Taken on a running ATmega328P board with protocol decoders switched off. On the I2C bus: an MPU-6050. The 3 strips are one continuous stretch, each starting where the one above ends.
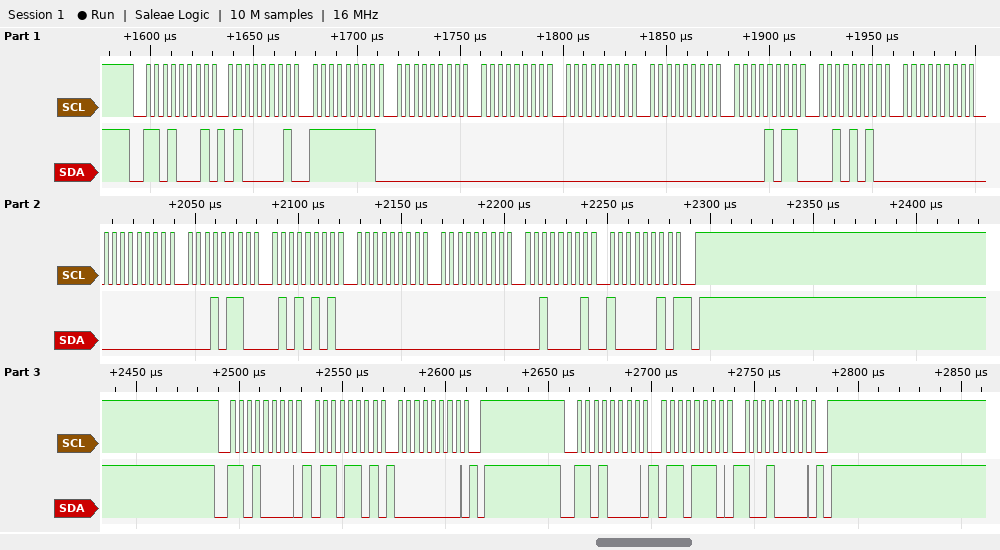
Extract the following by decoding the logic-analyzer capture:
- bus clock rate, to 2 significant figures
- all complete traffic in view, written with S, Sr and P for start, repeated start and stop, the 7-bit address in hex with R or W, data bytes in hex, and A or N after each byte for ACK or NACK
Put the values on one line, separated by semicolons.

250 kHz; S 68R A 41 A FF A 00 A 00 A 00 A 00 A 0B A 2A A 00 A 00 A 16 A 55 A 00 A 00 A 21 A 82 N P S 68W A 6D A 00 A P S 68W A 6E A 90 A P
